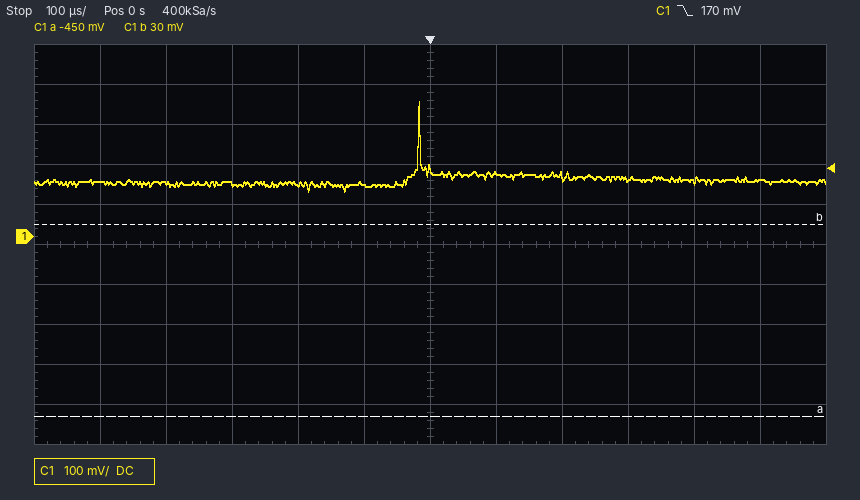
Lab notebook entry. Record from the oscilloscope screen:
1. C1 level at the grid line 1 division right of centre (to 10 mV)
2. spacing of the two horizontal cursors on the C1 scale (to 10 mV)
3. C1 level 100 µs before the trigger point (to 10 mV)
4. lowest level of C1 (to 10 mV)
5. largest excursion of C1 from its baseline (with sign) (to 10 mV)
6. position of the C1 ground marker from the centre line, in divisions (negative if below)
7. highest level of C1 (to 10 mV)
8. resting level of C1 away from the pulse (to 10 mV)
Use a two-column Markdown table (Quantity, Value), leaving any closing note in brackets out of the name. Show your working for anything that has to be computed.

| Quantity | Value |
|---|---|
| C1 level at the grid line 1 division right of centre | 160 mV |
| spacing of the two horizontal cursors on the C1 scale | 480 mV |
| C1 level 100 µs before the trigger point | 130 mV |
| lowest level of C1 | 110 mV |
| largest excursion of C1 from its baseline (with sign) | 340 mV − (140 mV) = +200 mV |
| position of the C1 ground marker from the centre line, in divisions | +0.2 div |
| highest level of C1 | 340 mV |
| resting level of C1 away from the pulse | 140 mV |
